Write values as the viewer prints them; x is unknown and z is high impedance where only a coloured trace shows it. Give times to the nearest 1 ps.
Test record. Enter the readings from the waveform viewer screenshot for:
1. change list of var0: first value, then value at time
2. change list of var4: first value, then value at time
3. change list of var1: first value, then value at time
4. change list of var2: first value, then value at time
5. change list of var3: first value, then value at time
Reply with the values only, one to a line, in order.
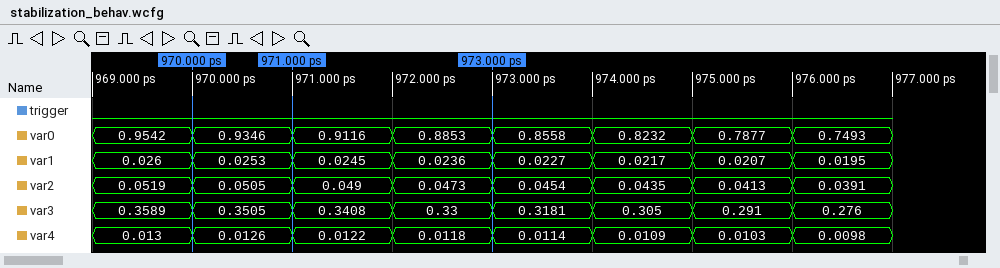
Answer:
0.9542, 0.9346 at 970 ps, 0.9116 at 971 ps, 0.8853 at 972 ps, 0.8558 at 973 ps, 0.8232 at 974 ps, 0.7877 at 975 ps, 0.7493 at 976 ps
0.013, 0.0126 at 970 ps, 0.0122 at 971 ps, 0.0118 at 972 ps, 0.0114 at 973 ps, 0.0109 at 974 ps, 0.0103 at 975 ps, 0.0098 at 976 ps
0.026, 0.0253 at 970 ps, 0.0245 at 971 ps, 0.0236 at 972 ps, 0.0227 at 973 ps, 0.0217 at 974 ps, 0.0207 at 975 ps, 0.0195 at 976 ps
0.0519, 0.0505 at 970 ps, 0.049 at 971 ps, 0.0473 at 972 ps, 0.0454 at 973 ps, 0.0435 at 974 ps, 0.0413 at 975 ps, 0.0391 at 976 ps
0.3589, 0.3505 at 970 ps, 0.3408 at 971 ps, 0.33 at 972 ps, 0.3181 at 973 ps, 0.305 at 974 ps, 0.291 at 975 ps, 0.276 at 976 ps
